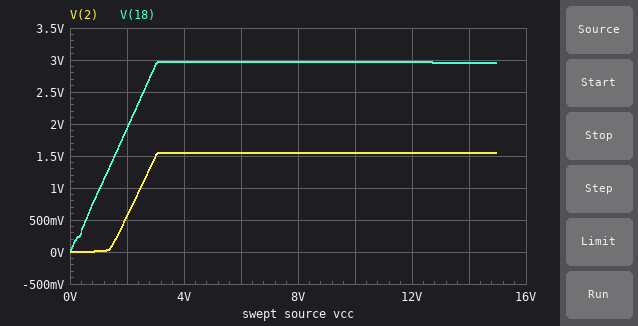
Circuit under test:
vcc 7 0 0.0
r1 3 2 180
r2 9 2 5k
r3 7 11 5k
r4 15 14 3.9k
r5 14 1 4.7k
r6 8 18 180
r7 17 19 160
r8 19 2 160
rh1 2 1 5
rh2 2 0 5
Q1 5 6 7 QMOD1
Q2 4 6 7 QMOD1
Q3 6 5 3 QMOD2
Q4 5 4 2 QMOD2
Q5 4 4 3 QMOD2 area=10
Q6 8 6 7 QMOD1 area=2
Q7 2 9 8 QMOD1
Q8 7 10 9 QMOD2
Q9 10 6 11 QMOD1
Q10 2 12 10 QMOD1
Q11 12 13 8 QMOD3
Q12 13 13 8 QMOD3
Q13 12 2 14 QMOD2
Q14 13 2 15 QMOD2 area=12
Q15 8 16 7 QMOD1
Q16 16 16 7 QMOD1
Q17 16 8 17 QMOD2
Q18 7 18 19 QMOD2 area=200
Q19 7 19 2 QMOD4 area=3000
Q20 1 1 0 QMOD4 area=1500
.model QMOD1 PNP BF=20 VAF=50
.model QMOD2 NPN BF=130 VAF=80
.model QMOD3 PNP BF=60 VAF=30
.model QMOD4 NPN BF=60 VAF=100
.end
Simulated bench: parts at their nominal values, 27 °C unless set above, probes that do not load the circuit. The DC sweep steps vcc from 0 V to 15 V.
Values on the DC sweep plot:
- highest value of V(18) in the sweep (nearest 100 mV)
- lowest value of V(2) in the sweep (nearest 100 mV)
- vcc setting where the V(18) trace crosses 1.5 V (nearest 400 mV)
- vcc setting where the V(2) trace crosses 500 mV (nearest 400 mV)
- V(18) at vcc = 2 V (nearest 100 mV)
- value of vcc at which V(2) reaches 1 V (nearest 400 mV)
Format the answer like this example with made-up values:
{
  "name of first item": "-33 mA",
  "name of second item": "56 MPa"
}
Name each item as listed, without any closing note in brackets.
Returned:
{
  "highest value of V(18) in the sweep": "3.0 V",
  "lowest value of V(2) in the sweep": "0 V",
  "vcc setting where the V(18) trace crosses 1.5 V": "1.6 V",
  "vcc setting where the V(2) trace crosses 500 mV": "2.0 V",
  "V(18) at vcc = 2 V": "1.9 V",
  "value of vcc at which V(2) reaches 1 V": "2.4 V"
}
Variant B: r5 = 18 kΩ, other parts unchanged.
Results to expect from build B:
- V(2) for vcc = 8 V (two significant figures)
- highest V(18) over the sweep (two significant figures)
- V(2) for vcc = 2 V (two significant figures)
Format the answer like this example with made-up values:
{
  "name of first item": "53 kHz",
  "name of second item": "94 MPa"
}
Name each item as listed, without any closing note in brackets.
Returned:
{
  "V(2) for vcc = 8 V": "2.0 V",
  "highest V(18) over the sweep": "3.4 V",
  "V(2) for vcc = 2 V": "560 mV"
}
